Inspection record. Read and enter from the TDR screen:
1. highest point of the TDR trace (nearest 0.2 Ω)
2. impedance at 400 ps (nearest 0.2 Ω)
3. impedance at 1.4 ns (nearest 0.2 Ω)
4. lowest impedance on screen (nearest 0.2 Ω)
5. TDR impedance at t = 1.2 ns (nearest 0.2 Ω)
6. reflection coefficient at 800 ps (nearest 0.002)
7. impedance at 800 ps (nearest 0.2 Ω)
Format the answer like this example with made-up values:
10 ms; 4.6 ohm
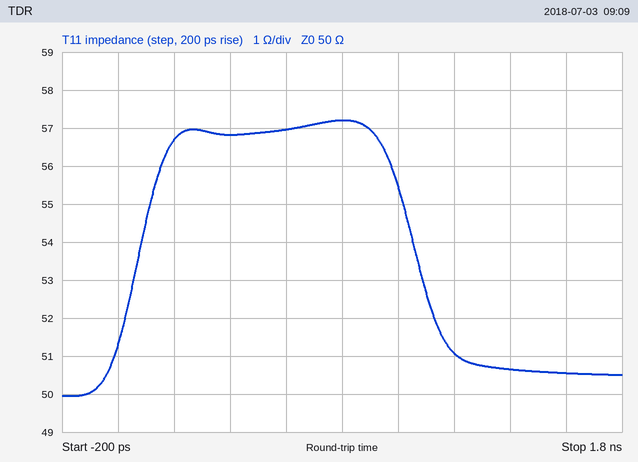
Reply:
57.2 Ω; 56.8 Ω; 50.6 Ω; 50.0 Ω; 51.0 Ω; +0.068; 57.2 Ω
